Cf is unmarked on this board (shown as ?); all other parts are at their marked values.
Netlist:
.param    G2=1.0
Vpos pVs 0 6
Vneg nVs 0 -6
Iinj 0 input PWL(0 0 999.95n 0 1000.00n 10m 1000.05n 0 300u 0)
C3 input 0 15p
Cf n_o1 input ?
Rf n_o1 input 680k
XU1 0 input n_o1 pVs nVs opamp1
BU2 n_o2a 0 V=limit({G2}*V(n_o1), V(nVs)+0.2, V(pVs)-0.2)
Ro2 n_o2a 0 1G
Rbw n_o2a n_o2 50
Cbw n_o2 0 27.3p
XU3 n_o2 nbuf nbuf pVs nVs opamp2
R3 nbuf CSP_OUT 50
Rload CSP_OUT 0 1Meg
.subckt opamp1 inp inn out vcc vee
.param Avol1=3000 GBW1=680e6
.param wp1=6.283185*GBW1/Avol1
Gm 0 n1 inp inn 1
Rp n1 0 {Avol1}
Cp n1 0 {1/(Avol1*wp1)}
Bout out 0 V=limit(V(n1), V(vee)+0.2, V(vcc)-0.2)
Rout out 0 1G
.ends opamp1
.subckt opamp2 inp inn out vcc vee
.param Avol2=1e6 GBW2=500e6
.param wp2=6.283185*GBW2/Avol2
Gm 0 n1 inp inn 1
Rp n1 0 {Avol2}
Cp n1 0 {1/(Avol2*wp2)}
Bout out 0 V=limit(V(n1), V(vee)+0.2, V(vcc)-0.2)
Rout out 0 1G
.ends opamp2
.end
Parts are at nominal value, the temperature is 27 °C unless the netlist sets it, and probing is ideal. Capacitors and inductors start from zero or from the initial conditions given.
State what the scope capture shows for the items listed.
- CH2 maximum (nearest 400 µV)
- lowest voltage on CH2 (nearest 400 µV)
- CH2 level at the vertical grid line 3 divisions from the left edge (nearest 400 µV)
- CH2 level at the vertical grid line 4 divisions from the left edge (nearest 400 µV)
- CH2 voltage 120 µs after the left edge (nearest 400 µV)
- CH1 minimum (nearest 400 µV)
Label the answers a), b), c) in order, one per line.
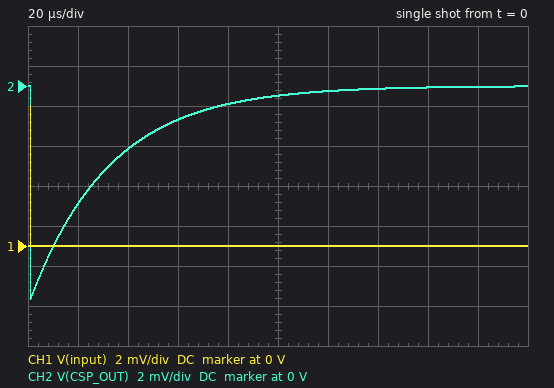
a) 0 V
b) -10.8 mV
c) -1.6 mV
d) -800 µV
e) -400 µV
f) 0 V
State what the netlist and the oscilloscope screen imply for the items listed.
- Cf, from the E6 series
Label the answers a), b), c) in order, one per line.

a) 47 pF
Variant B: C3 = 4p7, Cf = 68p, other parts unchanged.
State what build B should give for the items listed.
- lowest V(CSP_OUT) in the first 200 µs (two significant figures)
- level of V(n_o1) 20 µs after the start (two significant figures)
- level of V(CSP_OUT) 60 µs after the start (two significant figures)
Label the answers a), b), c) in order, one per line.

a) -7.4 mV
b) -4.9 mV
c) -2.1 mV
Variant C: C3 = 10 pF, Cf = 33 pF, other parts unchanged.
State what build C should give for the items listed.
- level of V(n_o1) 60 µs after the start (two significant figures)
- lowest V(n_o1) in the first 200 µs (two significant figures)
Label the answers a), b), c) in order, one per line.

a) -1.1 mV
b) -15 mV
